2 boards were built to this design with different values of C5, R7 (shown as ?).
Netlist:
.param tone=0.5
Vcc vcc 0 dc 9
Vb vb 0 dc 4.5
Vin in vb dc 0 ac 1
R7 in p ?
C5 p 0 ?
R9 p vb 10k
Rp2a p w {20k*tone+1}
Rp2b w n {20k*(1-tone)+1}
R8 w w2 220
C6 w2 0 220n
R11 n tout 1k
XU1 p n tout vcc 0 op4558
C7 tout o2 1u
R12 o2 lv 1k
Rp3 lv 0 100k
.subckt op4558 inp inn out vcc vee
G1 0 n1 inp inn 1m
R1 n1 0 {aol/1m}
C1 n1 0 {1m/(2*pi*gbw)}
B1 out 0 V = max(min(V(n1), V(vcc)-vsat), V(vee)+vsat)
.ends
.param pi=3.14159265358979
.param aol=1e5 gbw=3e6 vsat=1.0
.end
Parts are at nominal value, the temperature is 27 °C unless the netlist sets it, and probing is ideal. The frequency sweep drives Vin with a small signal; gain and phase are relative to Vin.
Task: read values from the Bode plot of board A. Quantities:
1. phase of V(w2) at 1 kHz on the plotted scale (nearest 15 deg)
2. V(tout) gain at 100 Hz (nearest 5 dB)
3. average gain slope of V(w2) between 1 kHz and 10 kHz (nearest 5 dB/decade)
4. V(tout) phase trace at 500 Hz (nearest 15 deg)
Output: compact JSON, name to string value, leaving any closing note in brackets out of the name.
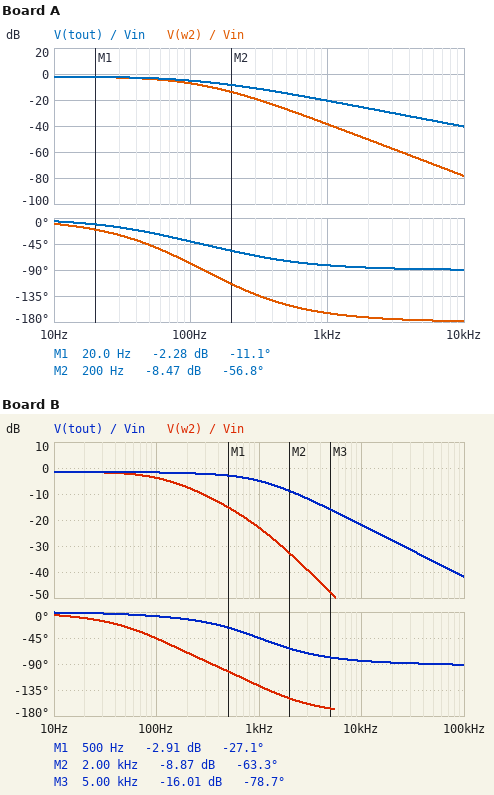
{"phase of V(w2) at 1 kHz on the plotted scale": "-165 deg", "V(tout) gain at 100 Hz": "-5 dB", "average gain slope of V(w2) between 1 kHz and 10 kHz": "-40 dB/decade", "V(tout) phase trace at 500 Hz": "-75 deg"}
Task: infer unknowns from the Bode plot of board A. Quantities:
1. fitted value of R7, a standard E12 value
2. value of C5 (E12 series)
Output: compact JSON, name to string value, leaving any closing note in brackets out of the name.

{"fitted value of R7, a standard E12 value": "2.7 kΩ", "value of C5": "680 nF"}
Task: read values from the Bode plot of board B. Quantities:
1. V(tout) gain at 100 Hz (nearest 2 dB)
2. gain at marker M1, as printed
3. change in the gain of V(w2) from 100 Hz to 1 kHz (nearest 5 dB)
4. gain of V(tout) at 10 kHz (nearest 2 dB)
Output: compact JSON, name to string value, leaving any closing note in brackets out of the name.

{"V(tout) gain at 100 Hz": "-2 dB", "gain at marker M1, as printed": "-2.91 dB", "change in the gain of V(w2) from 100 Hz to 1 kHz": "-20 dB", "gain of V(tout) at 10 kHz": "-22 dB"}
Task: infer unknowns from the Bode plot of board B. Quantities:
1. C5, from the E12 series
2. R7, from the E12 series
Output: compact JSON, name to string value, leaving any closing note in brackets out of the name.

{"C5, from the E12 series": "120 nF", "R7, from the E12 series": "1.8 kΩ"}
